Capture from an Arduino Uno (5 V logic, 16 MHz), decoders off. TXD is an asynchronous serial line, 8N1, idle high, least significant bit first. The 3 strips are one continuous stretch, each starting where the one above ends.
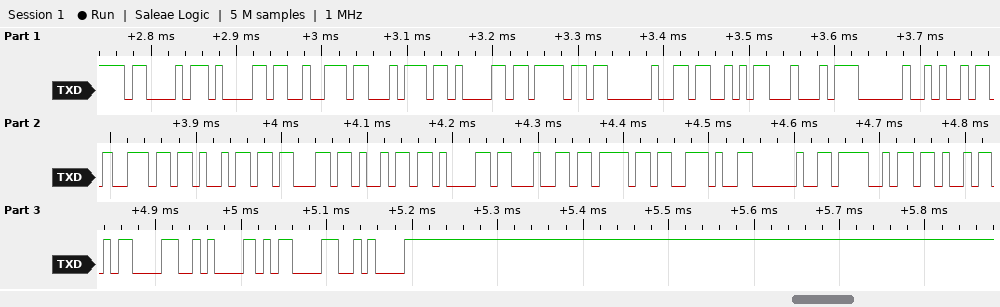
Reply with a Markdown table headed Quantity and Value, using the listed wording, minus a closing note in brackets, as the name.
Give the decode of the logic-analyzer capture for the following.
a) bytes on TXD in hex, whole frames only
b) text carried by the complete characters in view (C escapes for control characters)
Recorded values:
| Quantity | Value |
|---|---|
| bytes on TXD in hex, whole frames only | 43 61 72 74 61 6F 20 53 44 20 69 6E 69 63 69 61 64 6F 2E 20 4F 4B 0D 0A 0D 0A |
| text carried by the complete characters in view | "Cartao SD iniciado. OK\r\n\r\n" |
